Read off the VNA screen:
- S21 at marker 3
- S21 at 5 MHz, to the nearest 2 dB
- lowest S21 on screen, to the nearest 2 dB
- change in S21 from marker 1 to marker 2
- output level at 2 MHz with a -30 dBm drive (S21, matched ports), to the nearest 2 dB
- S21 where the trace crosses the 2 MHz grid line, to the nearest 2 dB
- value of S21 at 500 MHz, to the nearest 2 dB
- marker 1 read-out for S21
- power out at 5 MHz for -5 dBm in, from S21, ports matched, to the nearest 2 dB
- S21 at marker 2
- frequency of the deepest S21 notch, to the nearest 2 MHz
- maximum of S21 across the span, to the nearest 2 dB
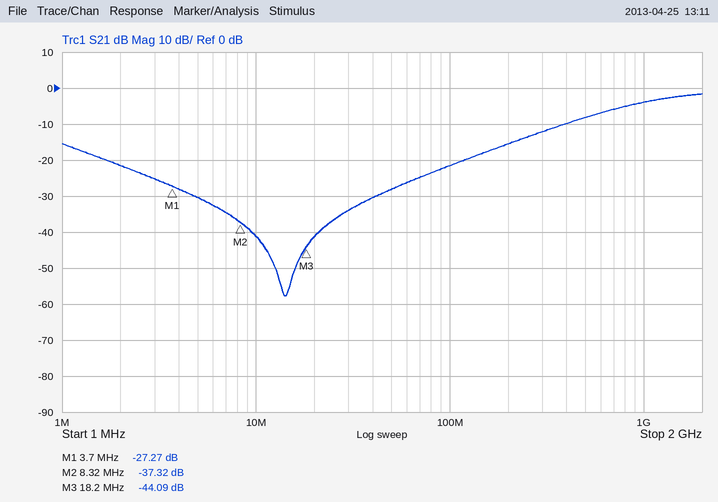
-44.09 dB
-30 dB
-58 dB
-10.05 dB
-52 dBm
-22 dB
-8 dB
-27.27 dB
-36 dBm
-37.32 dB
14 MHz
-2 dB
